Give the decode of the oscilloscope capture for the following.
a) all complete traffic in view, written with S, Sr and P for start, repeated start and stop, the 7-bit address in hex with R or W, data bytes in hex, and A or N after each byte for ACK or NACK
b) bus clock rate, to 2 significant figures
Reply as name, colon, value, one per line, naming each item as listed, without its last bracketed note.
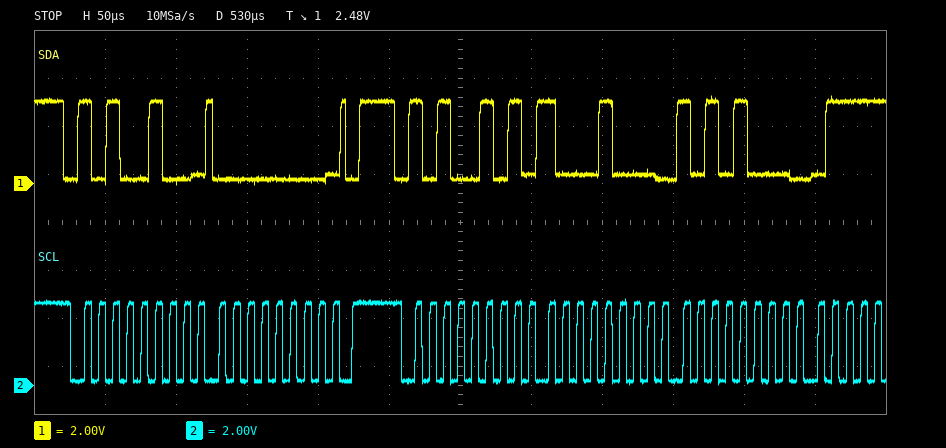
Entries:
all complete traffic in view, written with S, Sr and P for start, repeated start and stop, the 7-bit address in hex with R or W, data bytes in hex, and A or N after each byte for ACK or NACK: S 52W A 00 A P S 52R A 88 A A8 A
bus clock rate, to 2 significant figures: 100 kHz
